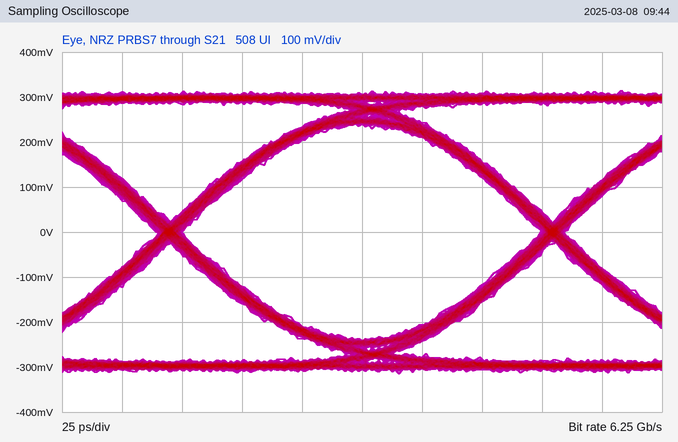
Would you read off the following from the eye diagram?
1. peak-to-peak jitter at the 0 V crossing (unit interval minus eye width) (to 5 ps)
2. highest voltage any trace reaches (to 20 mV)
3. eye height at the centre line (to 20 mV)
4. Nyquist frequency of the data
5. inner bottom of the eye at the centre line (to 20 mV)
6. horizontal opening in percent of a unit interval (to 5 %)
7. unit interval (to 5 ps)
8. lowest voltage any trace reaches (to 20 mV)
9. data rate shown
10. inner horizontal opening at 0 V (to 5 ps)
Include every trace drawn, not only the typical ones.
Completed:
10 ps
320 mV
480 mV
3.125 GHz
-240 mV
95 %
160 ps
-320 mV
6.25 Gb/s
150 ps
